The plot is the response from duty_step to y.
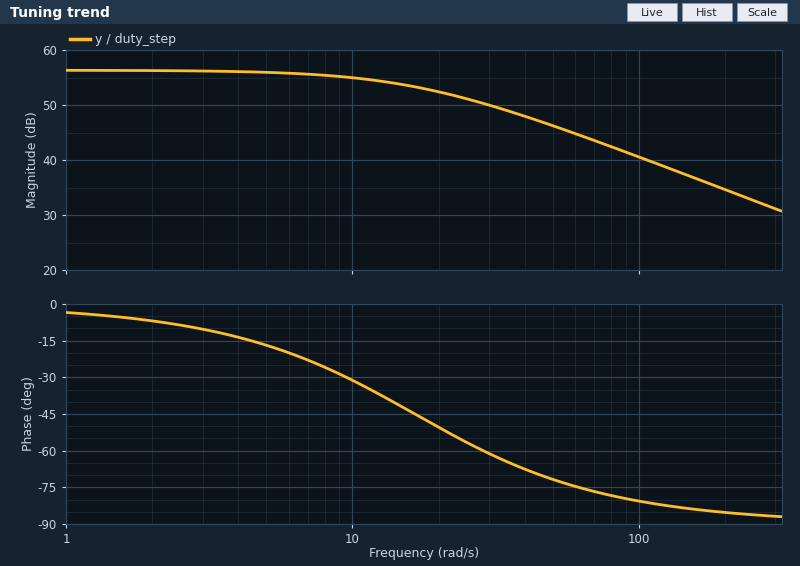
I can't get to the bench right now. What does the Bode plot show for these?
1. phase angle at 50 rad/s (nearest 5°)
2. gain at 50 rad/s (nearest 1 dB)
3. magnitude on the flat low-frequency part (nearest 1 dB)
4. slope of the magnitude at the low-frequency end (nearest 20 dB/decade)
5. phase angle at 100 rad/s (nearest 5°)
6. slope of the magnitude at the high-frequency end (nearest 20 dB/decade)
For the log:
-70°
46 dB
56 dB
0 dB/decade
-80°
-20 dB/decade
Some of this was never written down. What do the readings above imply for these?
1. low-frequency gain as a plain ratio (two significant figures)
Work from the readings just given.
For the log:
630
